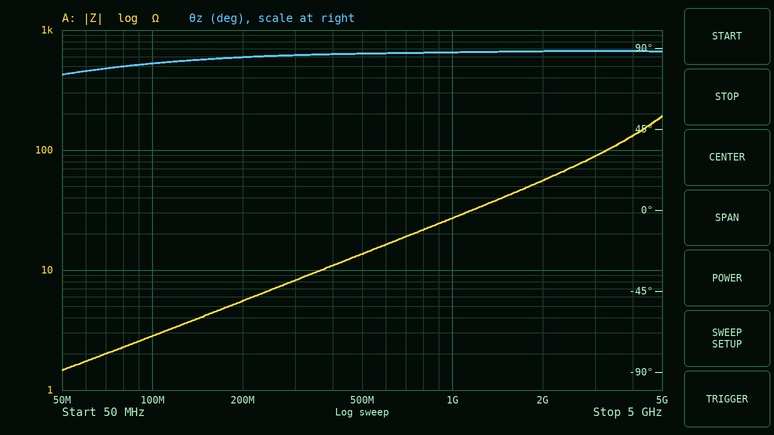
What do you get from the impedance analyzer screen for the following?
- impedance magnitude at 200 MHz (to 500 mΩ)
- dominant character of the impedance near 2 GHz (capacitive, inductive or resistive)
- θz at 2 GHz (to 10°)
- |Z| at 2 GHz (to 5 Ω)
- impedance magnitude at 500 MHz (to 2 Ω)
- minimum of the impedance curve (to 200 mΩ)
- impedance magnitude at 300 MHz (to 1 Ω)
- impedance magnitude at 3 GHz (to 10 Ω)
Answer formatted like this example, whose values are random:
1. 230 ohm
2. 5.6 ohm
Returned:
1. 5.5 Ω
2. inductive
3. 90°
4. 55 Ω
5. 14 Ω
6. 1.4 Ω
7. 8 Ω
8. 90 Ω
